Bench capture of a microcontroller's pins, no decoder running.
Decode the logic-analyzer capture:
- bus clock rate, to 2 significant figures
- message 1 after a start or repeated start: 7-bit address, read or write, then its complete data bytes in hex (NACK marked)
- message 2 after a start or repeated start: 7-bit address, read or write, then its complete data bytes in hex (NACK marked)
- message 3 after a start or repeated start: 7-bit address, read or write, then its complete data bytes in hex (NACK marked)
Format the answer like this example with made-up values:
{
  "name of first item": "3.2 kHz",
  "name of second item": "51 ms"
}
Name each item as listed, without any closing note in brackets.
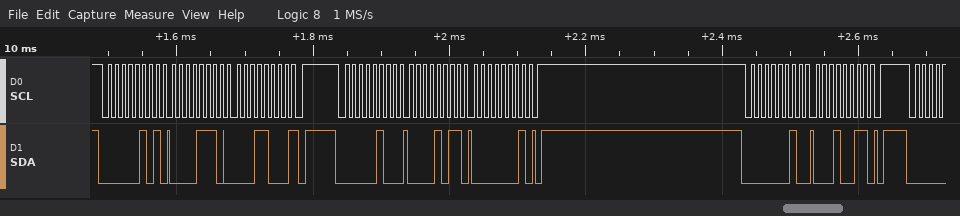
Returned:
{
  "bus clock rate, to 2 significant figures": "100 kHz",
  "message 1 after a start or repeated start: 7-bit address, read or write, then its complete data bytes in hex": "0x02 read: 0E 18 NACK",
  "message 2 after a start or repeated start: 7-bit address, read or write, then its complete data bytes in hex": "0x02 write: 0B 01",
  "message 3 after a start or repeated start: 7-bit address, read or write, then its complete data bytes in hex": "0x01 write: 13"
}
